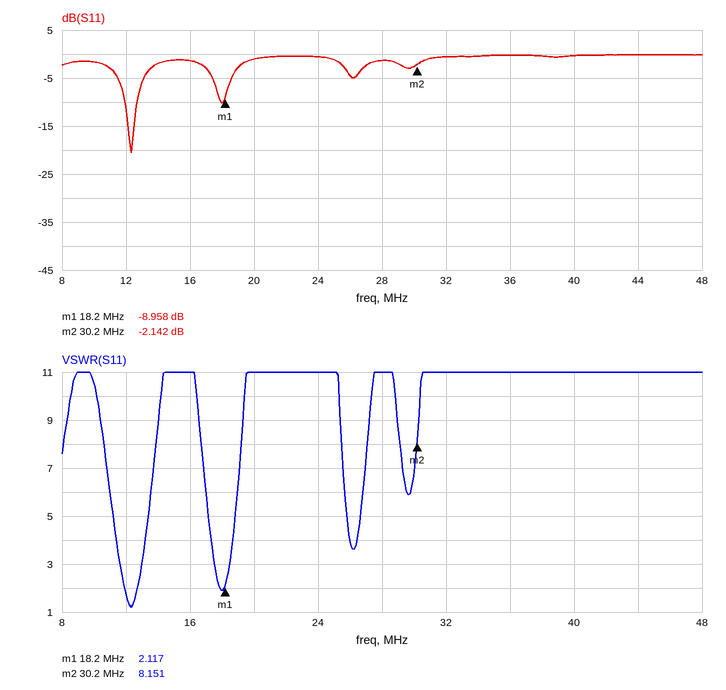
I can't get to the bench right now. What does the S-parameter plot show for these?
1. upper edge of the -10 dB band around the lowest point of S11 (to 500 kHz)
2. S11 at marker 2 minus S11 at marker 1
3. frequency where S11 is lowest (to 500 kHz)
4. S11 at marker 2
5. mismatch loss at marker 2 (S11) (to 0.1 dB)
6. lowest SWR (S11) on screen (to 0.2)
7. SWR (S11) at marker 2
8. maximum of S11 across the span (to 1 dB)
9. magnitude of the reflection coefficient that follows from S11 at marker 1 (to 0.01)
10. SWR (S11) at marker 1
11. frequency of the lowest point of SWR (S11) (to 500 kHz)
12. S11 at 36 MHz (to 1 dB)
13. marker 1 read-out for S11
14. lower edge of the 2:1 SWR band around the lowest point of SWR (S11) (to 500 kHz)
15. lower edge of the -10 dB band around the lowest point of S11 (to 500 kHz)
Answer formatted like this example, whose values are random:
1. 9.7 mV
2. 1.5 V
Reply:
1. 12.5 MHz
2. 6.816 dB
3. 12.5 MHz
4. -2.142 dB
5. 4.1 dB
6. 1.2
7. 8.151
8. 0 dB
9. 0.36
10. 2.117
11. 12.5 MHz
12. 0 dB
13. -8.958 dB
14. 12.0 MHz
15. 12.0 MHz
